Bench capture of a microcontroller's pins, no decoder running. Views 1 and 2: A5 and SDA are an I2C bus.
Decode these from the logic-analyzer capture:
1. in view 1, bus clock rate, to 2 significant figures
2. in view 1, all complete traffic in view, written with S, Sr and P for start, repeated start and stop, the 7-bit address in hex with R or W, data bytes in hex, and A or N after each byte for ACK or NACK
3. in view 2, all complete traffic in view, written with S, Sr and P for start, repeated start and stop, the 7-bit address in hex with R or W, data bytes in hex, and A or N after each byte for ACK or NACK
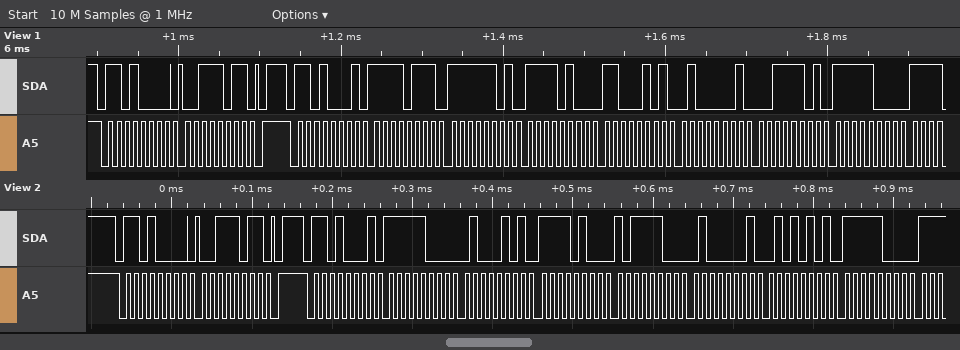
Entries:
100 kHz
S 68W A 3B A P S 68R A F7 A FD A F4 A C5 A 41 A 3D A F8 A
S 68W A 3B A P S 68R A F8 A 45 A F4 A BC A 41 A 55 A F8 A
